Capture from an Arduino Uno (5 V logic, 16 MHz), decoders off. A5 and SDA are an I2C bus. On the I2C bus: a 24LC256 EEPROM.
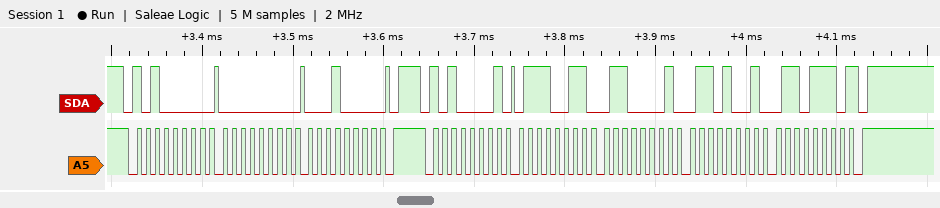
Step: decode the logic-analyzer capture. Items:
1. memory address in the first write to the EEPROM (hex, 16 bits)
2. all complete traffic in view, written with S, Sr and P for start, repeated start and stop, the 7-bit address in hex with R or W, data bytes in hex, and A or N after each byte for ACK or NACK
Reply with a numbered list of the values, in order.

1. 0x0010
2. S 50W A 00 A 10 A P S 50R A 73 A 61 A 69 A 6E N P
